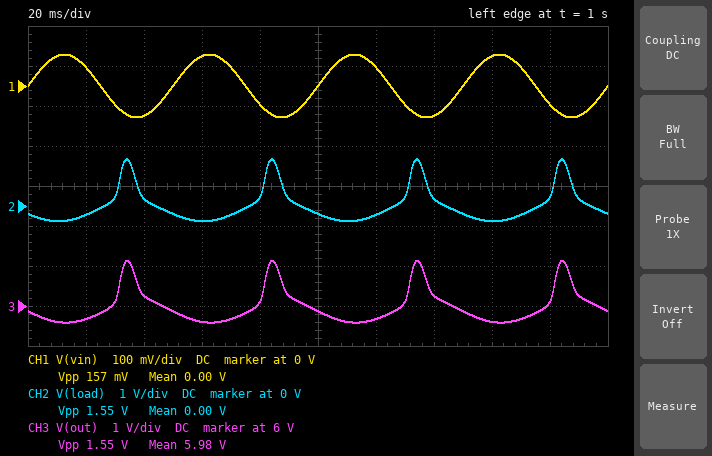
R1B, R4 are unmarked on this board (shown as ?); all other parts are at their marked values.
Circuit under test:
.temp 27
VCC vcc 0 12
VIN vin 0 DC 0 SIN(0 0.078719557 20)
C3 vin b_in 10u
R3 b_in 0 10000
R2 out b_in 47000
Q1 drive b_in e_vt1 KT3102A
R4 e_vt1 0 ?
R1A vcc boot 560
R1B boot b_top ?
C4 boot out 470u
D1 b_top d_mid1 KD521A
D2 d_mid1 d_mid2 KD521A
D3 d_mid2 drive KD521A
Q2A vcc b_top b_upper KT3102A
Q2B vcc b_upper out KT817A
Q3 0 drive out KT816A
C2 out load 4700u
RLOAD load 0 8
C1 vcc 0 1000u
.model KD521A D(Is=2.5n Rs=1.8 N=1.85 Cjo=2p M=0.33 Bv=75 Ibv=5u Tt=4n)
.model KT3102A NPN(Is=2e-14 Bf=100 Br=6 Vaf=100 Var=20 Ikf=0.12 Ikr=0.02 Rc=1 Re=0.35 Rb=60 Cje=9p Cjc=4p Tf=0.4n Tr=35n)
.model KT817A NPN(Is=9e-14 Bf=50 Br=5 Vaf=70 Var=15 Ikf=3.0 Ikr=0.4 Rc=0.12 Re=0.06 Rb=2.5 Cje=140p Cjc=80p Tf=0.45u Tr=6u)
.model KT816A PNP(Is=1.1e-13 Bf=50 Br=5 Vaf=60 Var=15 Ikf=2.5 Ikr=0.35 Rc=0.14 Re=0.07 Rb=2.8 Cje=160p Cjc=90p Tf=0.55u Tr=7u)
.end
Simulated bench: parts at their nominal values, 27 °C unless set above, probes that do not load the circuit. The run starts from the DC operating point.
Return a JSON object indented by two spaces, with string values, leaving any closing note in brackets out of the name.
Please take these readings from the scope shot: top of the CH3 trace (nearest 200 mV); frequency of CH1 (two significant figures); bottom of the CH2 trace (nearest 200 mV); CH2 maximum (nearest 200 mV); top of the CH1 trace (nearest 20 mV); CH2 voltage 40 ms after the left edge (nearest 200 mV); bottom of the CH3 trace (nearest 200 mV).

{
  "top of the CH3 trace": "7.2 V",
  "frequency of CH1": "20 Hz",
  "bottom of the CH2 trace": "-400 mV",
  "CH2 maximum": "1.2 V",
  "top of the CH1 trace": "80 mV",
  "CH2 voltage 40 ms after the left edge": "200 mV",
  "bottom of the CH3 trace": "5.6 V"
}
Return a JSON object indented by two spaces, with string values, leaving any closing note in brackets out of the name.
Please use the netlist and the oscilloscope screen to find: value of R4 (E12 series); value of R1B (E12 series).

{
  "value of R4": "120 Ω",
  "value of R1B": "2.7 kΩ"
}
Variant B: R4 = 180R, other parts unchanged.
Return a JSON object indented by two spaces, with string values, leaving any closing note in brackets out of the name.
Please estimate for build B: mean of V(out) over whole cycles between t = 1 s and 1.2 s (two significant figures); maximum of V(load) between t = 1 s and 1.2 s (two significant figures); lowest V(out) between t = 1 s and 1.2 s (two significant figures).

{
  "mean of V(out) over whole cycles between t = 1 s and 1.2 s": "6.3 V",
  "maximum of V(load) between t = 1 s and 1.2 s": "670 mV",
  "lowest V(out) between t = 1 s and 1.2 s": "6.0 V"
}
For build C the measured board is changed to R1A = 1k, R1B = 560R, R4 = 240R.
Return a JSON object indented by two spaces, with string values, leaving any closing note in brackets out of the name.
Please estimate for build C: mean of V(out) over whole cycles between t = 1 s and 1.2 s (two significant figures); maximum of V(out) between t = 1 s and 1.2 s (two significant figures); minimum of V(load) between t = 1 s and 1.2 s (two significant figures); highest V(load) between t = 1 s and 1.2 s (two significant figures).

{
  "mean of V(out) over whole cycles between t = 1 s and 1.2 s": "7.8 V",
  "maximum of V(out) between t = 1 s and 1.2 s": "8.0 V",
  "minimum of V(load) between t = 1 s and 1.2 s": "-160 mV",
  "highest V(load) between t = 1 s and 1.2 s": "190 mV"
}
